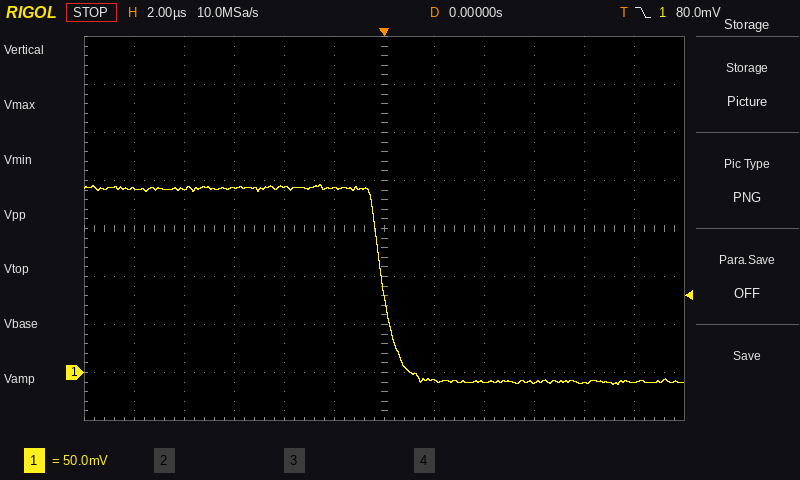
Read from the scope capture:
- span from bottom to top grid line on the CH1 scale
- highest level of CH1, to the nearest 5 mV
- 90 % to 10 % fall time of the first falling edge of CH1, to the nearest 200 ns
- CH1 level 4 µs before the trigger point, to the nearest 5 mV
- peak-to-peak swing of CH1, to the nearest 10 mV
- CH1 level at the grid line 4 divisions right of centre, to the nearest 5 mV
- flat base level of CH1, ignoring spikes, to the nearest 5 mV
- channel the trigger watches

400 mV
195 mV
1.2 µs
195 mV
210 mV
-10 mV
-10 mV
CH1
